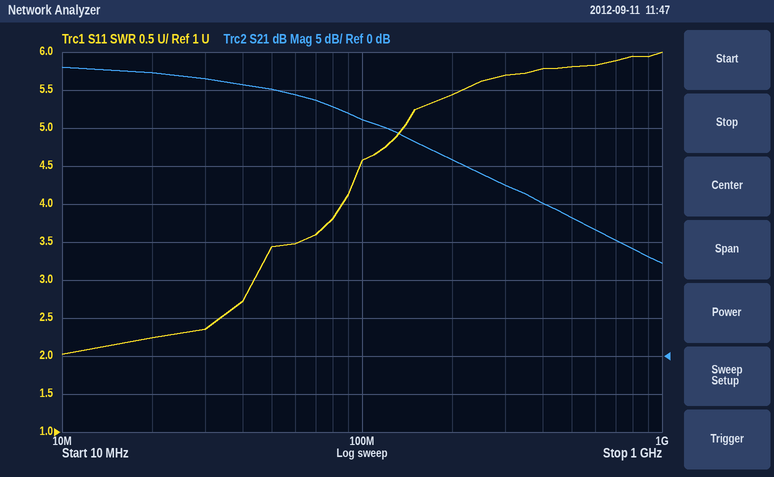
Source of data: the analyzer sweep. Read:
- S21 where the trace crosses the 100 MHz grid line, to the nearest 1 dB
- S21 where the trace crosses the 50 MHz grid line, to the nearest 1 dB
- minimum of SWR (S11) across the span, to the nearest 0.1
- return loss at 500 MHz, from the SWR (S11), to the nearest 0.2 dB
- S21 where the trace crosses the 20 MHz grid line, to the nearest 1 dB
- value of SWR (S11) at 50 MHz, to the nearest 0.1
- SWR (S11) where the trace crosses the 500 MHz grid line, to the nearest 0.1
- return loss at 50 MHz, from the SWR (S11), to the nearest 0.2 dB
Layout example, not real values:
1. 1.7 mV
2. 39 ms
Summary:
1. 31 dB
2. 35 dB
3. 2.0
4. 3.0 dB
5. 37 dB
6. 3.4
7. 5.8
8. 5.2 dB
